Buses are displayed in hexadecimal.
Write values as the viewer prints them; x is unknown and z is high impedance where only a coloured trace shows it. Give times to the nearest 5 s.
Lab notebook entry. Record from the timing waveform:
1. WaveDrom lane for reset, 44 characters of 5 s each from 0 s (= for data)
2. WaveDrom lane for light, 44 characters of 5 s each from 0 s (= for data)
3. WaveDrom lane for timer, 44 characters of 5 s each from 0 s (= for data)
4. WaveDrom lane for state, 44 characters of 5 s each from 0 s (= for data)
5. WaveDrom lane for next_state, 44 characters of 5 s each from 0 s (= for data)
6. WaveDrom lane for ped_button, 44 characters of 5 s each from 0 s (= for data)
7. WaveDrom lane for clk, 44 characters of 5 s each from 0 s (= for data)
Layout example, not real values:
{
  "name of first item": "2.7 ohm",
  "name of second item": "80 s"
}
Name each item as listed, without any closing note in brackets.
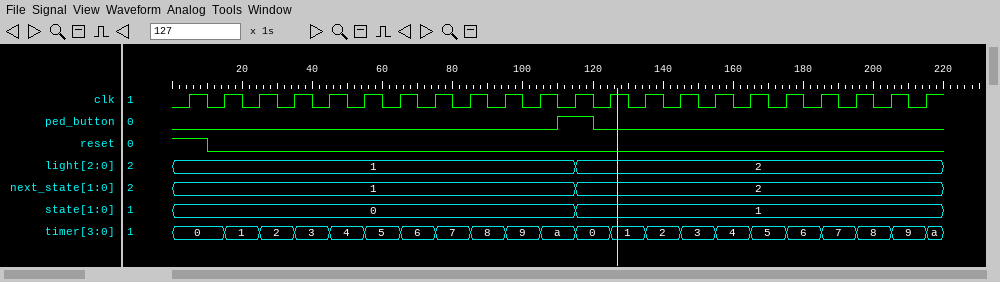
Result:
{
  "WaveDrom lane for reset, 44 characters of 5 s each from 0 s": "{name: 'reset', wave: '1.0.........................................'}",
  "WaveDrom lane for light, 44 characters of 5 s each from 0 s": "{name: 'light', wave: '=......................=....................', data: '1 2'}",
  "WaveDrom lane for timer, 44 characters of 5 s each from 0 s": "{name: 'timer', wave: '=..=.=.=.=.=.=.=.=.=.=.=.=.=.=.=.=.=.=.=.=.=', data: '0 1 2 3 4 5 6 7 8 9 a 0 1 2 3 4 5 6 7 8 9 a'}",
  "WaveDrom lane for state, 44 characters of 5 s each from 0 s": "{name: 'state', wave: '=......................=....................', data: '0 1'}",
  "WaveDrom lane for next_state, 44 characters of 5 s each from 0 s": "{name: 'next_state', wave: '=......................=....................', data: '1 2'}",
  "WaveDrom lane for ped_button, 44 characters of 5 s each from 0 s": "{name: 'ped_button', wave: '0.....................1.0...................'}",
  "WaveDrom lane for clk, 44 characters of 5 s each from 0 s": "{name: 'clk', wave: '01010101010101010101010101010101010101010101'}"
}
